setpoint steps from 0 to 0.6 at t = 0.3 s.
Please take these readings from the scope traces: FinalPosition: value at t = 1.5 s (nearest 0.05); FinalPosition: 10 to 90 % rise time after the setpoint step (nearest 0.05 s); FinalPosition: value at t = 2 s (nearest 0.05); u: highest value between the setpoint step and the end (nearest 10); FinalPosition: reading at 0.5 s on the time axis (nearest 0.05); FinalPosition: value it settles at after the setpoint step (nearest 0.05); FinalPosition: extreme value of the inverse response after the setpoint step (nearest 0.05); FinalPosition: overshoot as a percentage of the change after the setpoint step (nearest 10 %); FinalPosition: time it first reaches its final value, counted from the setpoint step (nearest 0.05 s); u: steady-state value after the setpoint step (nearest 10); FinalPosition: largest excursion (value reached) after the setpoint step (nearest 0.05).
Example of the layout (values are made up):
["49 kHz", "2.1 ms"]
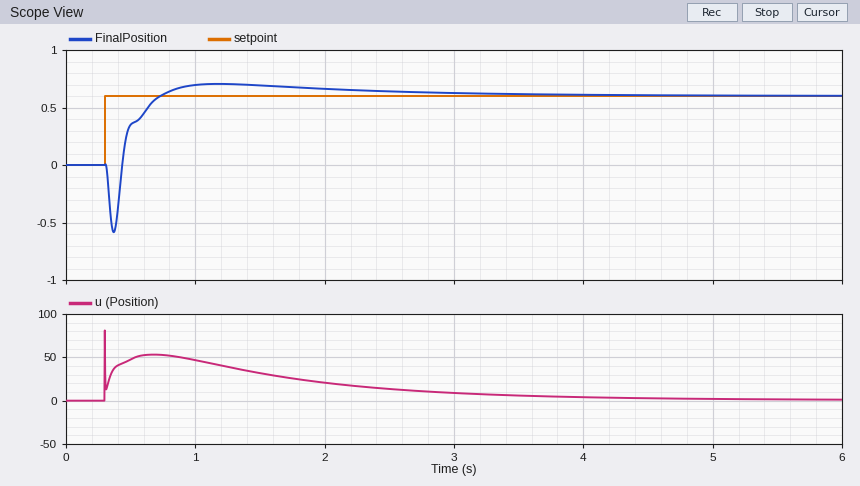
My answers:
["0.70", "0.20 s", "0.65", "80", "0.35", "0.60", "-0.60", "20 %", "0.45 s", "0", "0.70"]
